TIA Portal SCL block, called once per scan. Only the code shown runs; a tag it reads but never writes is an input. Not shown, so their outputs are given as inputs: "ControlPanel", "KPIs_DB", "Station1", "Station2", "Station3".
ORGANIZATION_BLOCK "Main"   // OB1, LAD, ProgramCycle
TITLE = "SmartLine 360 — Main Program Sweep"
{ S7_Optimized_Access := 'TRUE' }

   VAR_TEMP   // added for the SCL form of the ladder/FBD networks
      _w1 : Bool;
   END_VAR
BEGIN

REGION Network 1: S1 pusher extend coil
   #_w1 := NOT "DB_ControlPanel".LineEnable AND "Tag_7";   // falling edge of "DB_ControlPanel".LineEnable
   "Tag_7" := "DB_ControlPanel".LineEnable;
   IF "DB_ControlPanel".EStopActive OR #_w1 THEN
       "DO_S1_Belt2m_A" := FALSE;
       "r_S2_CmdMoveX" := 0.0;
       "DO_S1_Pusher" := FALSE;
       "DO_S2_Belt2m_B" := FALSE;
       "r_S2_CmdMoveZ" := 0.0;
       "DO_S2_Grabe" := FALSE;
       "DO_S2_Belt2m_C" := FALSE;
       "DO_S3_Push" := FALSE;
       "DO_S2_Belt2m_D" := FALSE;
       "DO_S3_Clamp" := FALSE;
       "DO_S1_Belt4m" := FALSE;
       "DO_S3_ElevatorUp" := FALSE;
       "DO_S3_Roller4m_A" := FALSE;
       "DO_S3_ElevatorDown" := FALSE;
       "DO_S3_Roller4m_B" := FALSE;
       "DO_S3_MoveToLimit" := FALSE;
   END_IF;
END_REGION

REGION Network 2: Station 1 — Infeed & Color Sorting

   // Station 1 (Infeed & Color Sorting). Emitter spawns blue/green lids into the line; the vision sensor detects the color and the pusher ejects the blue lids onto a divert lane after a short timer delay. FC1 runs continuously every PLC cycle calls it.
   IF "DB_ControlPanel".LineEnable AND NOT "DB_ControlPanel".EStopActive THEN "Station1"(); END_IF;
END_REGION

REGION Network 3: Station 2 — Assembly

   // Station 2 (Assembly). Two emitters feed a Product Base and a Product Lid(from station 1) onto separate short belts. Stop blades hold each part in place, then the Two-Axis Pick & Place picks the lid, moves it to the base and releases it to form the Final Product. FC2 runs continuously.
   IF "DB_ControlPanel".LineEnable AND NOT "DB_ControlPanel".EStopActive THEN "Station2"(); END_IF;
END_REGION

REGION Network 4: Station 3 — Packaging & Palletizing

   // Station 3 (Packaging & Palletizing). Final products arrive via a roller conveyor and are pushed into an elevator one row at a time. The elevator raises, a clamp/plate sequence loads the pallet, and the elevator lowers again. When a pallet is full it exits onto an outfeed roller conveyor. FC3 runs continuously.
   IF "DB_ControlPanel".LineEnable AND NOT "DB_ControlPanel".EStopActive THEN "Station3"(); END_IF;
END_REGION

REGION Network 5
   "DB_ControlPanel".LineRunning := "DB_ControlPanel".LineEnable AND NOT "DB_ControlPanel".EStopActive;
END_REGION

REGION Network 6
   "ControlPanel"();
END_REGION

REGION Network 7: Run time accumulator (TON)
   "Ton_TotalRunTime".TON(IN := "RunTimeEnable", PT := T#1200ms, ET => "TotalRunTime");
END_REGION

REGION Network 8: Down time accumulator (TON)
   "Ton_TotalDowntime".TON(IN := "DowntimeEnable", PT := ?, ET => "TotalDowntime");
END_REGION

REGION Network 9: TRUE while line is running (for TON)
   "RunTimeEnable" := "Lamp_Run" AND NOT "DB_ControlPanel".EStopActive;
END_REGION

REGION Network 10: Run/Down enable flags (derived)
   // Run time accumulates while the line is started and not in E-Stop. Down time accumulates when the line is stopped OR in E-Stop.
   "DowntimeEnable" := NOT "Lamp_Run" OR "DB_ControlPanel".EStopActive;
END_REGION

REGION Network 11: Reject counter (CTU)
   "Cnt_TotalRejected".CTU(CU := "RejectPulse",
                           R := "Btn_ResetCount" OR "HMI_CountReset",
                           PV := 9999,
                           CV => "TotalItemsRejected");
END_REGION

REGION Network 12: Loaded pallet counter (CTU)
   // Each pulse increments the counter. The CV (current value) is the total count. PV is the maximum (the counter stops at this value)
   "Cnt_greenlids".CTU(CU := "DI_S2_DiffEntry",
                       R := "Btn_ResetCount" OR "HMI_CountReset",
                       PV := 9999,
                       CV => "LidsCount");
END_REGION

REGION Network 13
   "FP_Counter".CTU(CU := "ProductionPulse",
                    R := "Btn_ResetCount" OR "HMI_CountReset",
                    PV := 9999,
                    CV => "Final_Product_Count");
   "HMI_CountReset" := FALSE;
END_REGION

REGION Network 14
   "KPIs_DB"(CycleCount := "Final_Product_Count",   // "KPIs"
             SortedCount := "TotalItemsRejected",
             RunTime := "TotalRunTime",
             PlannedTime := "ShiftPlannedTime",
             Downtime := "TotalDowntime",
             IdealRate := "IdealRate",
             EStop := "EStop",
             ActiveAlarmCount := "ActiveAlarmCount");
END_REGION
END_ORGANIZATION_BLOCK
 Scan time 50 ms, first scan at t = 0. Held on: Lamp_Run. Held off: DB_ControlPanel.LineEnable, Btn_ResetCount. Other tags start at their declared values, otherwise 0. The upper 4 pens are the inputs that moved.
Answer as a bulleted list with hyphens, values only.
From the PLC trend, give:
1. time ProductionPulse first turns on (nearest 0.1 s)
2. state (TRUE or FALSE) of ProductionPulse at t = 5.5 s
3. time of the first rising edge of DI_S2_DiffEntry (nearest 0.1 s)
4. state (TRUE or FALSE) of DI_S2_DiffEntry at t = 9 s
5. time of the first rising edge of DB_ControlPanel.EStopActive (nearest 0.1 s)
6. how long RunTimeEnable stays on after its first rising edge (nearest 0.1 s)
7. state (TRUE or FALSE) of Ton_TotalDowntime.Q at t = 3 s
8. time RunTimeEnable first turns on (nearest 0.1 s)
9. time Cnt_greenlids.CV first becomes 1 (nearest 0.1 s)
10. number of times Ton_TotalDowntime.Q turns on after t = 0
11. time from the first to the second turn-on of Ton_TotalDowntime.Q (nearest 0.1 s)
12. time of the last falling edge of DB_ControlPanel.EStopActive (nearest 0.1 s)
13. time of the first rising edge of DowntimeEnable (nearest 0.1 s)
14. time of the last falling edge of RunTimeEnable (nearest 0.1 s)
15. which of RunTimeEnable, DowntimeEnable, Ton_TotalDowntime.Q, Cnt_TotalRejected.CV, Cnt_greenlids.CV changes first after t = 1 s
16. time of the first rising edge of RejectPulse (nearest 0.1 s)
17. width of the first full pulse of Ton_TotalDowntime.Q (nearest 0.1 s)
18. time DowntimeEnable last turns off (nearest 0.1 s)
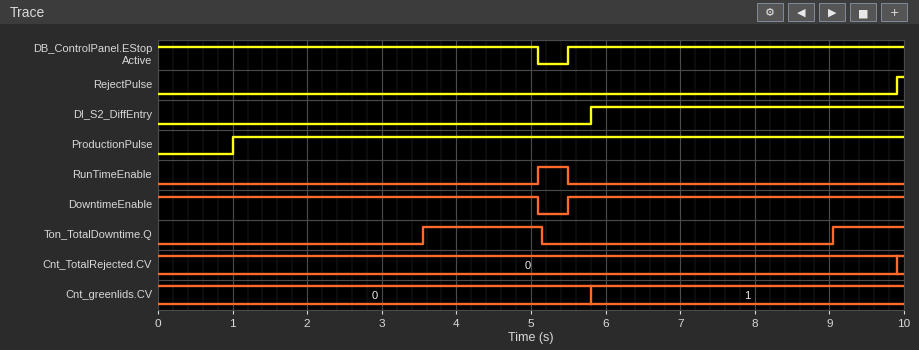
- 1.0 s
- TRUE
- 5.8 s
- TRUE
- 5.5 s
- 0.4 s
- FALSE
- 5.1 s
- 5.8 s
- 2
- 5.5 s
- 5.1 s
- 5.5 s
- 5.5 s
- Ton_TotalDowntime.Q
- 9.9 s
- 1.6 s
- 5.1 s
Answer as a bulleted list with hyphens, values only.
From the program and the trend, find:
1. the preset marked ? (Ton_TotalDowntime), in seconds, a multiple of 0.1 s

- 3.5 s
